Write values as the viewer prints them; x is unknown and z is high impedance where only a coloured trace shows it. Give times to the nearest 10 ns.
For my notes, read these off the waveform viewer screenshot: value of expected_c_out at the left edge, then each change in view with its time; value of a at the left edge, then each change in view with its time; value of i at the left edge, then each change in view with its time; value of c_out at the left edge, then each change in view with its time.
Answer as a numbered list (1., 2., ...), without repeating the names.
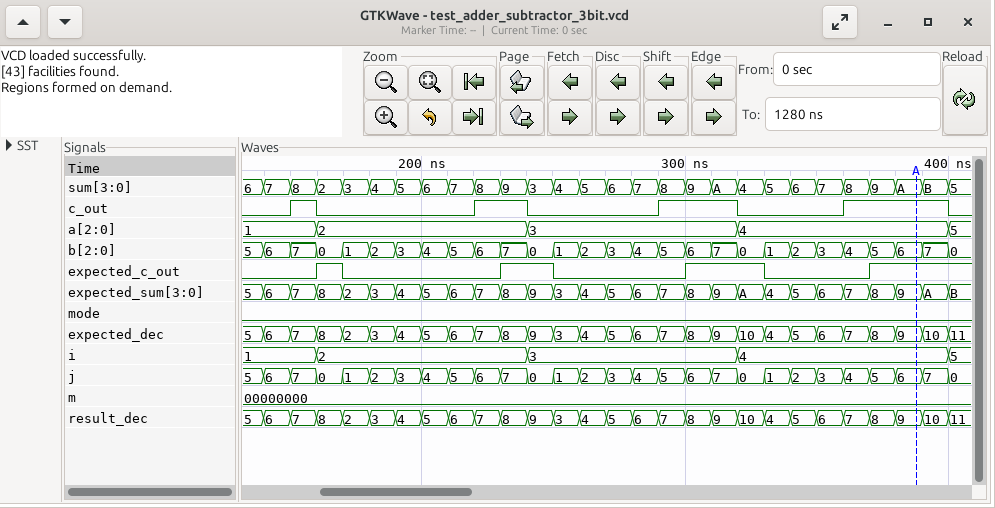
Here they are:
1. 0, 1 at 160 ns, 0 at 170 ns, 1 at 230 ns, 0 at 250 ns, 1 at 300 ns, 0 at 330 ns, 1 at 370 ns
2. 1, 2 at 160 ns, 3 at 240 ns, 4 at 320 ns, 5 at 400 ns
3. 1, 2 at 160 ns, 3 at 240 ns, 4 at 320 ns, 5 at 400 ns
4. 0, 1 at 150 ns, 0 at 160 ns, 1 at 220 ns, 0 at 240 ns, 1 at 290 ns, 0 at 320 ns, 1 at 360 ns, 0 at 400 ns
